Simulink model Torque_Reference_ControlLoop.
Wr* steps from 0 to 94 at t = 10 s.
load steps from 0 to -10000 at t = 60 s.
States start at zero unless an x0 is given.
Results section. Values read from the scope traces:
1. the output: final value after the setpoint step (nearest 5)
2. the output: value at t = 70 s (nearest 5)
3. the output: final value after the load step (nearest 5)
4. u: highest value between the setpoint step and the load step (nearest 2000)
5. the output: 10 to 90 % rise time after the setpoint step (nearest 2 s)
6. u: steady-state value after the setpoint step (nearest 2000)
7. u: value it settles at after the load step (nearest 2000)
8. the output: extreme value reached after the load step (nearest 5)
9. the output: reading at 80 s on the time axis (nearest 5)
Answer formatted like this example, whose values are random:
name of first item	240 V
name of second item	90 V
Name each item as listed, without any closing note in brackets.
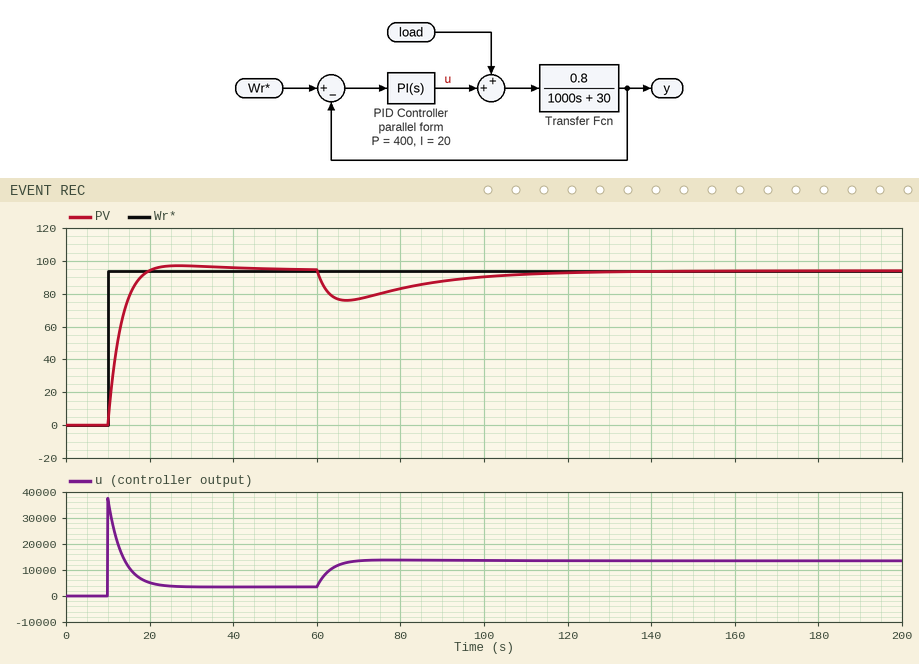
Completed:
the output: final value after the setpoint step	95
the output: value at t = 70 s	75
the output: final value after the load step	95
u: highest value between the setpoint step and the load step	38000
the output: 10 to 90 % rise time after the setpoint step	6 s
u: steady-state value after the setpoint step	4000
u: value it settles at after the load step	14000
the output: extreme value reached after the load step	75
the output: reading at 80 s on the time axis	85
